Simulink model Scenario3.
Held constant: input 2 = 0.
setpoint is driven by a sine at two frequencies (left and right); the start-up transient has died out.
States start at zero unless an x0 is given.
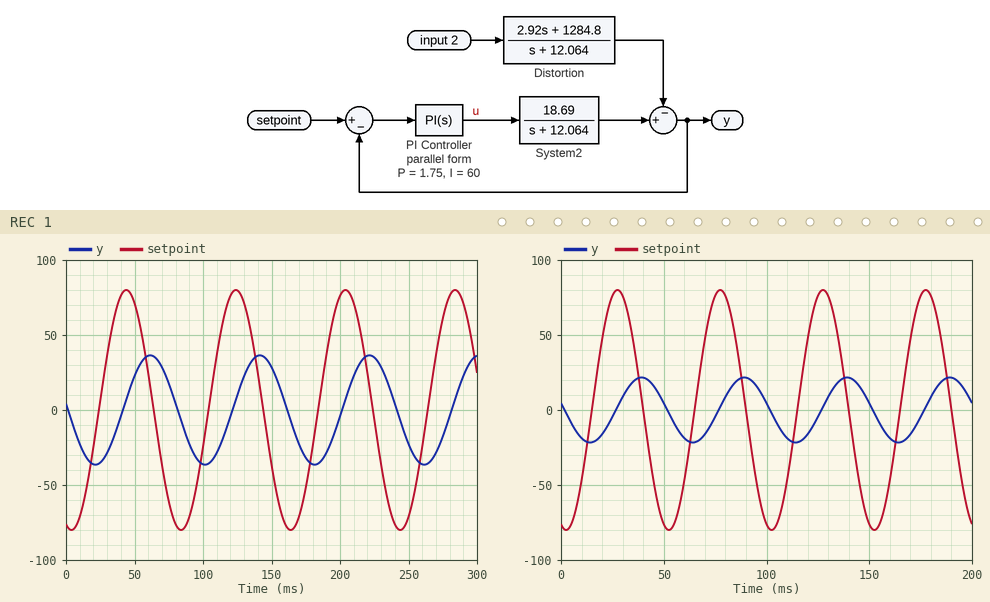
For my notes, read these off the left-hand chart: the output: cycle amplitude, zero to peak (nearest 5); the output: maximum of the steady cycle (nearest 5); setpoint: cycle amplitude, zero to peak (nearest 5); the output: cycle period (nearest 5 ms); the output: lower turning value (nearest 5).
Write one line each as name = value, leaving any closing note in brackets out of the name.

the output: cycle amplitude, zero to peak = 35
the output: maximum of the steady cycle = 35
setpoint: cycle amplitude, zero to peak = 80
the output: cycle period = 80 ms
the output: lower turning value = -35
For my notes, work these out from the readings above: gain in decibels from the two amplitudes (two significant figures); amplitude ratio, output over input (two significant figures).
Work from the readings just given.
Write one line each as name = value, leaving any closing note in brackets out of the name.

gain in decibels from the two amplitudes = -7.2 dB
amplitude ratio, output over input = 0.44
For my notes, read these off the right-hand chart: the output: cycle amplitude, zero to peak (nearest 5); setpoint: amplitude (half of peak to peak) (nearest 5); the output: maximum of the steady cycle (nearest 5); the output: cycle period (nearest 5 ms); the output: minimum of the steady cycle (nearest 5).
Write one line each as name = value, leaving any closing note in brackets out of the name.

the output: cycle amplitude, zero to peak = 20
setpoint: amplitude (half of peak to peak) = 80
the output: maximum of the steady cycle = 20
the output: cycle period = 50 ms
the output: minimum of the steady cycle = -20
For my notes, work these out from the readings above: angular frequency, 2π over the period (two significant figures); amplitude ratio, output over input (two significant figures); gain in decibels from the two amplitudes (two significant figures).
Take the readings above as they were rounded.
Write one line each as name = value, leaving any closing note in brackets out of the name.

angular frequency, 2π over the period = 0.13 rad/ms
amplitude ratio, output over input = 0.25
gain in decibels from the two amplitudes = -12 dB
